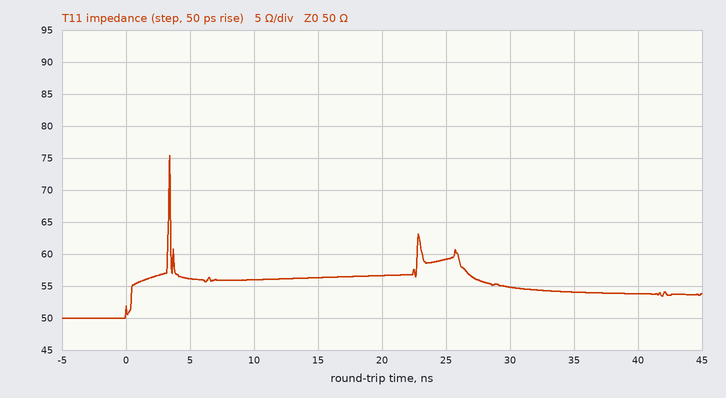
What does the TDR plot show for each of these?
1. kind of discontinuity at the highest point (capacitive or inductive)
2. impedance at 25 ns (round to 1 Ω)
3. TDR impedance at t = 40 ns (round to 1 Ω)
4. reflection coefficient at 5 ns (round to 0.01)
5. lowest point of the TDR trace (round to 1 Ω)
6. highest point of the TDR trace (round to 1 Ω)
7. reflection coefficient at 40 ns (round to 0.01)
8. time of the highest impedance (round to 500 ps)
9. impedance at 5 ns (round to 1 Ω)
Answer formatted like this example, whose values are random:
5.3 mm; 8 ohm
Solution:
inductive; 59 Ω; 54 Ω; +0.06; 50 Ω; 75 Ω; +0.04; 3.5 ns; 56 Ω
